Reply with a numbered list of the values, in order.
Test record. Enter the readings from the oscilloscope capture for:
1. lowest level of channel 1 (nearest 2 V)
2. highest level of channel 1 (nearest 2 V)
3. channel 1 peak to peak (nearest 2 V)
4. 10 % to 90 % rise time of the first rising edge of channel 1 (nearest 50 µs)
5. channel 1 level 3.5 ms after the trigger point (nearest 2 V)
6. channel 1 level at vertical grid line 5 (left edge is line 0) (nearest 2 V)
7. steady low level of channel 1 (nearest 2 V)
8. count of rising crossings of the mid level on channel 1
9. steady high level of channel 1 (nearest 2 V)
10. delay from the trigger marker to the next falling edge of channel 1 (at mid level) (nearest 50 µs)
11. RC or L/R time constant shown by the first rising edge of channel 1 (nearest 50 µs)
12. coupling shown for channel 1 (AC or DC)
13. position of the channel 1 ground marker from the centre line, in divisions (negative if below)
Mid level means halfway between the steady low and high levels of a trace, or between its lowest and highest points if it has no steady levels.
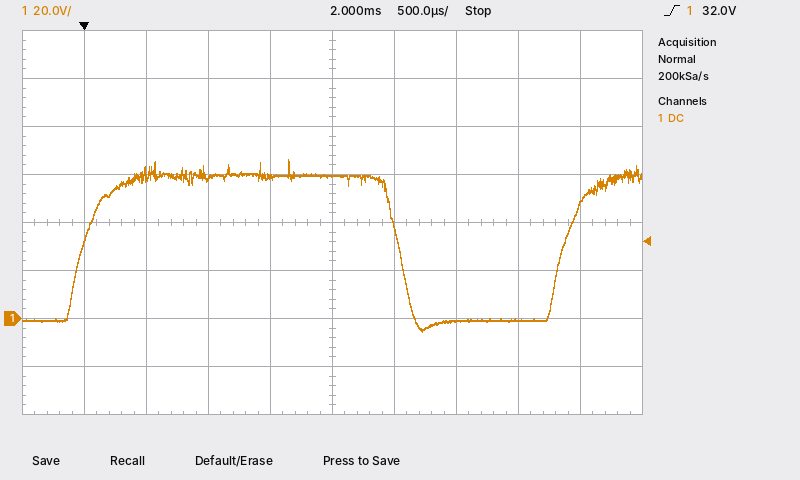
1. -6 V
2. 66 V
3. 72 V
4. 350 µs
5. 0 V
6. 60 V
7. 0 V
8. 2
9. 60 V
10. 2.55 ms
11. 150 µs
12. DC
13. -2.0 div
